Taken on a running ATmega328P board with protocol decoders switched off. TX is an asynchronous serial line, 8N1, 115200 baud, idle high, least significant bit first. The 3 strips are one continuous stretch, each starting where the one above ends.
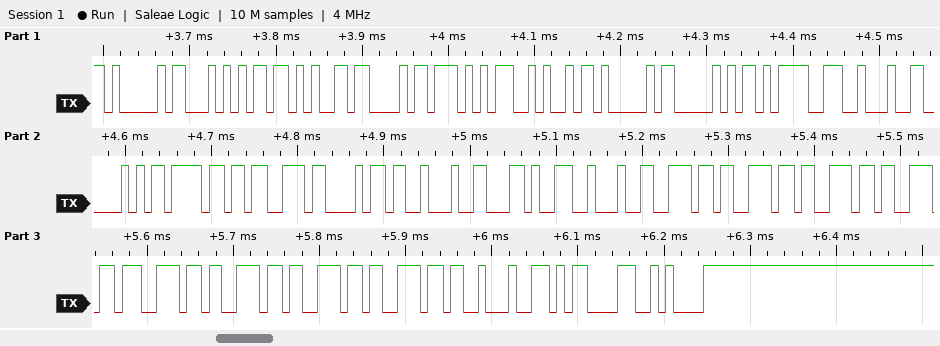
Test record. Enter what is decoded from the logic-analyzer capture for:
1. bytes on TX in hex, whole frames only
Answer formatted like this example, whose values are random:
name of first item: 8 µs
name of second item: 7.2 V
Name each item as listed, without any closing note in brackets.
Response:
bytes on TX in hex, whole frames only: 41 54 2B 43 57 4A 41 50 3D 22 50 6F 73 68 22 2C 22 6E 6E 6E 6E 6E 6E 6E 6E 22 0D 0A
